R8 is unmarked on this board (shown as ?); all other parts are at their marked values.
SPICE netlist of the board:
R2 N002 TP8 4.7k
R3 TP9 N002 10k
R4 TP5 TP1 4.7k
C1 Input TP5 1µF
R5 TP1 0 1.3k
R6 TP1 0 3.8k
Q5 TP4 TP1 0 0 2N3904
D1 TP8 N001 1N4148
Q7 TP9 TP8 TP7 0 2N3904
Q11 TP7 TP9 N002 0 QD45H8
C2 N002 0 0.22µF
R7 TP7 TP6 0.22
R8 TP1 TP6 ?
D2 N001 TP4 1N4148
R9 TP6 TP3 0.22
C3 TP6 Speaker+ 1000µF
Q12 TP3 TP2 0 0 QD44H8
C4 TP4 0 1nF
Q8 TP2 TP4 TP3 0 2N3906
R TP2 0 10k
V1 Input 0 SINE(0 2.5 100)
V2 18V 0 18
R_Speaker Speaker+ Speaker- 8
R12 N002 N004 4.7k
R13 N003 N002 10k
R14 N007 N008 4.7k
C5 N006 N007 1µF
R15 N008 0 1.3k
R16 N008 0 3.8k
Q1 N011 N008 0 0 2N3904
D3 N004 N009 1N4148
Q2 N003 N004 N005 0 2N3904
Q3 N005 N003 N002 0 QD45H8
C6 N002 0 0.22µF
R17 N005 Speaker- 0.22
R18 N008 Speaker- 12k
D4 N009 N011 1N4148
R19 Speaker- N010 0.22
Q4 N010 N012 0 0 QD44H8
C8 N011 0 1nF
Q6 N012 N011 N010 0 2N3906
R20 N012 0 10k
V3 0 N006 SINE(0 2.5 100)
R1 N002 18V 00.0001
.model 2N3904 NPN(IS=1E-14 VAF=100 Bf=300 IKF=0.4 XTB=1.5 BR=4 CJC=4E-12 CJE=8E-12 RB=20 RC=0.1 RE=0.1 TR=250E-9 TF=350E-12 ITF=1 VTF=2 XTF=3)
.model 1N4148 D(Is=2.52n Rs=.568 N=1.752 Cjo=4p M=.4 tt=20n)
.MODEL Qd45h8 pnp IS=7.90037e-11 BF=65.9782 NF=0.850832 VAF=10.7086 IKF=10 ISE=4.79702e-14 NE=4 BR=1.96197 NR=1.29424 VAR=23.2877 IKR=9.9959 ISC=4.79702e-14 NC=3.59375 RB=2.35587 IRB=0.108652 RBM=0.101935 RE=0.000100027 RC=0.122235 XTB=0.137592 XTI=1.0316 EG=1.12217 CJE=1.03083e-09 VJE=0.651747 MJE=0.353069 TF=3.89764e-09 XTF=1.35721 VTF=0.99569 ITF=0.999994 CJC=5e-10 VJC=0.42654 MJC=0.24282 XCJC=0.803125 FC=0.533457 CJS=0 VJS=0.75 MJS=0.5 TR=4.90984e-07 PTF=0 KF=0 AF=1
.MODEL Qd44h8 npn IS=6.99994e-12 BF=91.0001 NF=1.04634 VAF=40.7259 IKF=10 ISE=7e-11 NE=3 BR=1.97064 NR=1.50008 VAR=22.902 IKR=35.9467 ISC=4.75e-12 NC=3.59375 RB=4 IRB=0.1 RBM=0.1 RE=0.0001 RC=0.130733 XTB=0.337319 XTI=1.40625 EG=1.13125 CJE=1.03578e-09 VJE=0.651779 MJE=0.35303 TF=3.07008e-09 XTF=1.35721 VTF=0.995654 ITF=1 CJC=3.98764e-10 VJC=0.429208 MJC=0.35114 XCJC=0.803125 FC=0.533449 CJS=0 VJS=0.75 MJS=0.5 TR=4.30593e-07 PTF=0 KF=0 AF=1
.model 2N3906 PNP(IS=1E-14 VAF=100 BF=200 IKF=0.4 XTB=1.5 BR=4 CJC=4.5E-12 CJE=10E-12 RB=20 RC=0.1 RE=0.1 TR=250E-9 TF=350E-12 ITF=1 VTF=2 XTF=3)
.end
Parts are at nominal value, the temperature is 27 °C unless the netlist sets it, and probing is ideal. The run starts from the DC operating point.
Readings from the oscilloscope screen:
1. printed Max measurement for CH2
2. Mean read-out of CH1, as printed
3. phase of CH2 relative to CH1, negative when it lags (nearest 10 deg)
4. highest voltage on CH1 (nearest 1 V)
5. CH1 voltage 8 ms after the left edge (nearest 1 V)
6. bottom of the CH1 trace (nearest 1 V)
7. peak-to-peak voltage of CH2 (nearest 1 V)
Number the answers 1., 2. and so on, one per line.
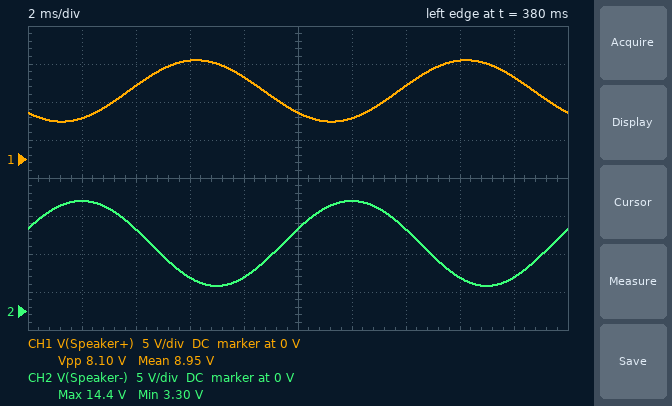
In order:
1. 14.4 V
2. 8.95 V
3. 150 deg
4. 13 V
5. 11 V
6. 5 V
7. 11 V
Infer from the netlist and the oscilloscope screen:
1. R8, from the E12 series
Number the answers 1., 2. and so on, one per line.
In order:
1. 8.2 kΩ
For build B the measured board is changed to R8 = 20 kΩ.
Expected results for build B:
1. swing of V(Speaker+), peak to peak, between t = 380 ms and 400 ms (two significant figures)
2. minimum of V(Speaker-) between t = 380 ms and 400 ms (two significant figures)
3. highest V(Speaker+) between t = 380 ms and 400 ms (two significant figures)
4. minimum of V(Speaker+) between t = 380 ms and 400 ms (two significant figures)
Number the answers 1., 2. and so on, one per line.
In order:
1. 13 V
2. 3.3 V
3. 15 V
4. 1.8 V
